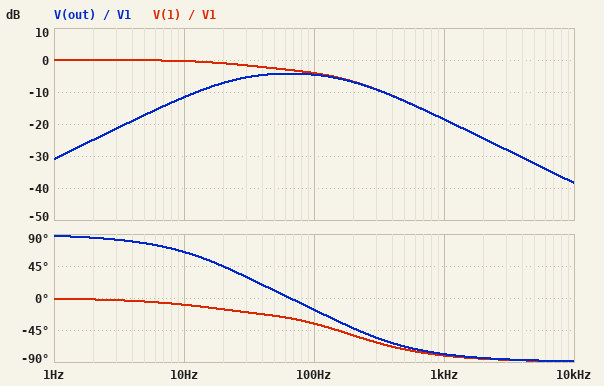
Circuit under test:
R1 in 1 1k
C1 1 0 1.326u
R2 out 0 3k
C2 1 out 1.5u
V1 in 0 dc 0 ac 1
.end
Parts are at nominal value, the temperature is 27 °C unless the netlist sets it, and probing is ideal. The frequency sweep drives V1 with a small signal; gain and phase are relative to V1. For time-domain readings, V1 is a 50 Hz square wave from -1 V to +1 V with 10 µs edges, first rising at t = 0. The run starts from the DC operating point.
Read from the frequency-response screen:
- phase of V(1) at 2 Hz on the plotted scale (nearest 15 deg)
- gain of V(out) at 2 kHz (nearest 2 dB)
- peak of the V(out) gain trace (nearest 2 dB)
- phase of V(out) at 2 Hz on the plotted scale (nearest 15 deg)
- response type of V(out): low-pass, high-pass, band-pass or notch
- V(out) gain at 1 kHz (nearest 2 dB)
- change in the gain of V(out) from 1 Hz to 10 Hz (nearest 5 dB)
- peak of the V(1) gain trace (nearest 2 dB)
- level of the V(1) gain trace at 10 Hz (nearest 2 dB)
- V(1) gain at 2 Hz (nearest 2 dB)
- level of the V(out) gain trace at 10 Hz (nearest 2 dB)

0 deg
-24 dB
-4 dB
90 deg
band-pass
-18 dB
20 dB
0 dB
0 dB
0 dB
-12 dB
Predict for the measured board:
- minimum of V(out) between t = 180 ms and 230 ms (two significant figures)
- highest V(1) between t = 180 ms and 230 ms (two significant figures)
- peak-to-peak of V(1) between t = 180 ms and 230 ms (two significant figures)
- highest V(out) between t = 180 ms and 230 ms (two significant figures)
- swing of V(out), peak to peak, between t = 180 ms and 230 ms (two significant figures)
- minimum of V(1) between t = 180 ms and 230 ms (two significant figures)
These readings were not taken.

-810 mV
880 mV
1.8 V
810 mV
1.6 V
-880 mV
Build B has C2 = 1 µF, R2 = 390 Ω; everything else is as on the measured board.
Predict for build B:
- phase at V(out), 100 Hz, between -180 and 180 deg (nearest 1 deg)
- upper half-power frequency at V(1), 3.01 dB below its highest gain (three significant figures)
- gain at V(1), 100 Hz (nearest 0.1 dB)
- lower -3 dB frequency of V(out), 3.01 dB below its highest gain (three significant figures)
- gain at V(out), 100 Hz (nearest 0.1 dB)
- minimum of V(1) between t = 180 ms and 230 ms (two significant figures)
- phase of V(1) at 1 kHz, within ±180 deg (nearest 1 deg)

25 deg
64.5 Hz
-5.2 dB
55.0 Hz
-17.7 dB
-970 mV
-71 deg
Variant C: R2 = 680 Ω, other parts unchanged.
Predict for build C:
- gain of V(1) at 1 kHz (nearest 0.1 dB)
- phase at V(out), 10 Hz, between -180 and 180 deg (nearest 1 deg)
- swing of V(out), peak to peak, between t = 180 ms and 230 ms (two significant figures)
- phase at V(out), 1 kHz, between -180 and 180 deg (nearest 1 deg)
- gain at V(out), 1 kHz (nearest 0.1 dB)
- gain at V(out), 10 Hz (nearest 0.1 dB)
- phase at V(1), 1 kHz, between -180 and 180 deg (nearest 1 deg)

-19.0 dB
76 deg
840 mV
-65 deg
-19.1 dB
-24.1 dB
-74 deg
